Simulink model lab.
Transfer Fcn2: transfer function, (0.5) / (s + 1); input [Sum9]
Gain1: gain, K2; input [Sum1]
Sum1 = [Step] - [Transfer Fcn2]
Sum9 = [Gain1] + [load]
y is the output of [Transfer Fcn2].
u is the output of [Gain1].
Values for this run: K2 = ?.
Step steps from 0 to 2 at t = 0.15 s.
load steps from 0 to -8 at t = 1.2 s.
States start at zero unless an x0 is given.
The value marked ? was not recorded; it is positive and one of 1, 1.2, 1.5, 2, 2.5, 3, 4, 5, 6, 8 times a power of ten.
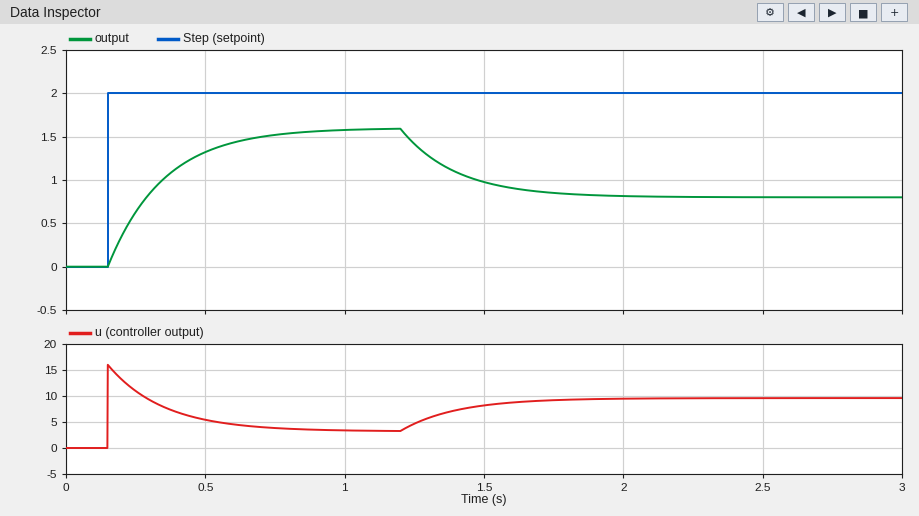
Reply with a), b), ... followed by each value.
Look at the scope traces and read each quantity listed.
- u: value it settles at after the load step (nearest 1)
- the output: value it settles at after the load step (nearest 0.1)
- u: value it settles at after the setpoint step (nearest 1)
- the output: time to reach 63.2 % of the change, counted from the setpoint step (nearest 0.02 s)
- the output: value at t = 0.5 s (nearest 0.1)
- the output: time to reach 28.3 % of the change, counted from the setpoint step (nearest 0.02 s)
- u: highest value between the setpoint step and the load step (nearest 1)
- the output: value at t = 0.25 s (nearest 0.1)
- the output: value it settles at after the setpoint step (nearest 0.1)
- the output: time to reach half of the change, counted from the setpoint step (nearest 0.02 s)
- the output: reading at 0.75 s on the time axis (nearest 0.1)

a) 10
b) 0.8
c) 3
d) 0.20 s
e) 1.3
f) 0.06 s
g) 16
h) 0.6
i) 1.6
j) 0.14 s
k) 1.5
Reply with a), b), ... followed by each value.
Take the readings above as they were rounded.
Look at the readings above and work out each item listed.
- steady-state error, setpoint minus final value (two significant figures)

a) 0.40
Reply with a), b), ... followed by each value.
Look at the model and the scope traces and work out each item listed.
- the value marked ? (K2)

a) 8
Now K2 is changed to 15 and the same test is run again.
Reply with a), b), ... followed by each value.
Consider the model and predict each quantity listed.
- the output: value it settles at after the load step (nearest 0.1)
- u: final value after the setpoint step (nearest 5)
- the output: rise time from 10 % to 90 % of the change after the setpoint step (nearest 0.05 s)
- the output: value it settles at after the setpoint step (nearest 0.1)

a) 1.3
b) 5
c) 0.25 s
d) 1.8
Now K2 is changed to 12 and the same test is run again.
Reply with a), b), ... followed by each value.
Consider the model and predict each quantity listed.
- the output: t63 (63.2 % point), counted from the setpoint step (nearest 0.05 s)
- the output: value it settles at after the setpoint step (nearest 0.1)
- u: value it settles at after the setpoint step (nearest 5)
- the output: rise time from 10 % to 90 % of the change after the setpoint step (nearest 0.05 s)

a) 0.15 s
b) 1.7
c) 5
d) 0.30 s
